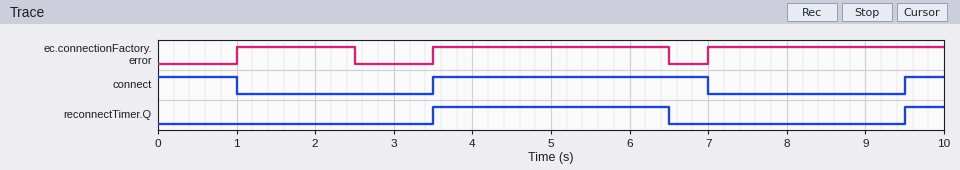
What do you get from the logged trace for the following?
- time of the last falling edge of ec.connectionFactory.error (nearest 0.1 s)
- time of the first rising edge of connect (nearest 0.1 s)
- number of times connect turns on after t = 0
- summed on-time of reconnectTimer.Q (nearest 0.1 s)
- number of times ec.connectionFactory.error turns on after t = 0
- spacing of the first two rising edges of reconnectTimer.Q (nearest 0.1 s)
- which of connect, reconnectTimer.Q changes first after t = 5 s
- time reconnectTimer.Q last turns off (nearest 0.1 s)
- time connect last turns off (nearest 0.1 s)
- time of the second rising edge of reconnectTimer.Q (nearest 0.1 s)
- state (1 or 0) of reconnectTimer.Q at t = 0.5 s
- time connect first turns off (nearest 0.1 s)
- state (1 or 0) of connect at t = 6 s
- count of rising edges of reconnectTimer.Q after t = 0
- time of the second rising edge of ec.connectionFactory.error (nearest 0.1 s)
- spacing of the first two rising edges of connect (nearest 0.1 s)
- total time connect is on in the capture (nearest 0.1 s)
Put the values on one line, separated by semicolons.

6.5 s; 3.5 s; 2; 3.5 s; 3; 6.0 s; reconnectTimer.Q; 6.5 s; 7.0 s; 9.5 s; 0; 1.0 s; 1; 2; 3.5 s; 6.0 s; 5.0 s
